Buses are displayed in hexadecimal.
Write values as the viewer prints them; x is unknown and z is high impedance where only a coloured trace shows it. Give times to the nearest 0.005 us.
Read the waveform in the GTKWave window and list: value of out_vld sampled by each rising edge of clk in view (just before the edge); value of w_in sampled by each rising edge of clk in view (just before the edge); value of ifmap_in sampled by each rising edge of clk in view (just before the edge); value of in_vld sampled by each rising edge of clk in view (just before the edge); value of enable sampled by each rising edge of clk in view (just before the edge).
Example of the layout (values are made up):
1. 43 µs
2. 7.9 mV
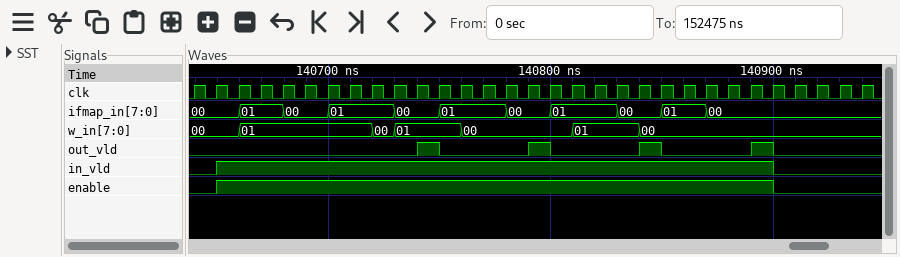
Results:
1. 0 0 0 0 0 0 0 0 0 0 0 1 0 0 0 0 1 0 0 0 0 1 0 0 0 0 1 0 0 0 0
2. 00, 00, 00, 01, 01, 01, 01, 01, 01, 00, 01, 01, 01, 00, 00, 00, 00, 00, 01, 01, 01, 00, 00, 00, 00, 00, 00, 00, 00, 00, 00
3. 00, 00, 00, 01, 01, 00, 00, 01, 01, 01, 00, 00, 01, 01, 01, 00, 00, 01, 01, 01, 00, 00, 01, 01, 00, 00, 00, 00, 00, 00, 00
4. 0 0 1 1 1 1 1 1 1 1 1 1 1 1 1 1 1 1 1 1 1 1 1 1 1 1 1 0 0 0 0
5. 0 0 1 1 1 1 1 1 1 1 1 1 1 1 1 1 1 1 1 1 1 1 1 1 1 1 1 0 0 0 0
